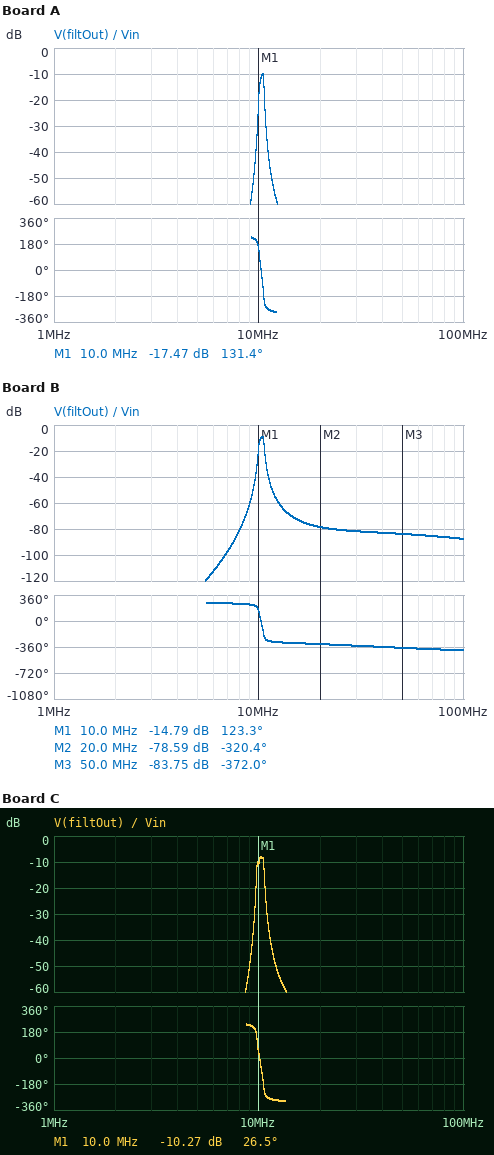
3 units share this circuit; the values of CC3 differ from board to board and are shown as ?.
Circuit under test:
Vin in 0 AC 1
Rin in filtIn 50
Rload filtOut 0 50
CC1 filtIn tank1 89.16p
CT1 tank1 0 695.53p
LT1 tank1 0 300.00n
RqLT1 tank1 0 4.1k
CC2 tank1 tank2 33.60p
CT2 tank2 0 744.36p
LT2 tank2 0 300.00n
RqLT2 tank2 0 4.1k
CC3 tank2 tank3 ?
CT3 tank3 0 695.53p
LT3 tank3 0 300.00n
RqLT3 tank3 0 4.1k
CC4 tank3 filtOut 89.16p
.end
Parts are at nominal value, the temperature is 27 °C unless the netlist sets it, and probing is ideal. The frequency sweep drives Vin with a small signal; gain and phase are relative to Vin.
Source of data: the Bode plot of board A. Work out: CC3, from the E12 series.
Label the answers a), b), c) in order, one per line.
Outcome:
a) 15 pF
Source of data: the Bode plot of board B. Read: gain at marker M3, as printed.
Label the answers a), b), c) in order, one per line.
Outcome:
a) -83.75 dB
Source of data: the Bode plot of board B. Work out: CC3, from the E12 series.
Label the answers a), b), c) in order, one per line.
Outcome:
a) 18 pF
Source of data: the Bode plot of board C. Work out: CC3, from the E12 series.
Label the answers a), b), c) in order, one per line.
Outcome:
a) 47 pF
